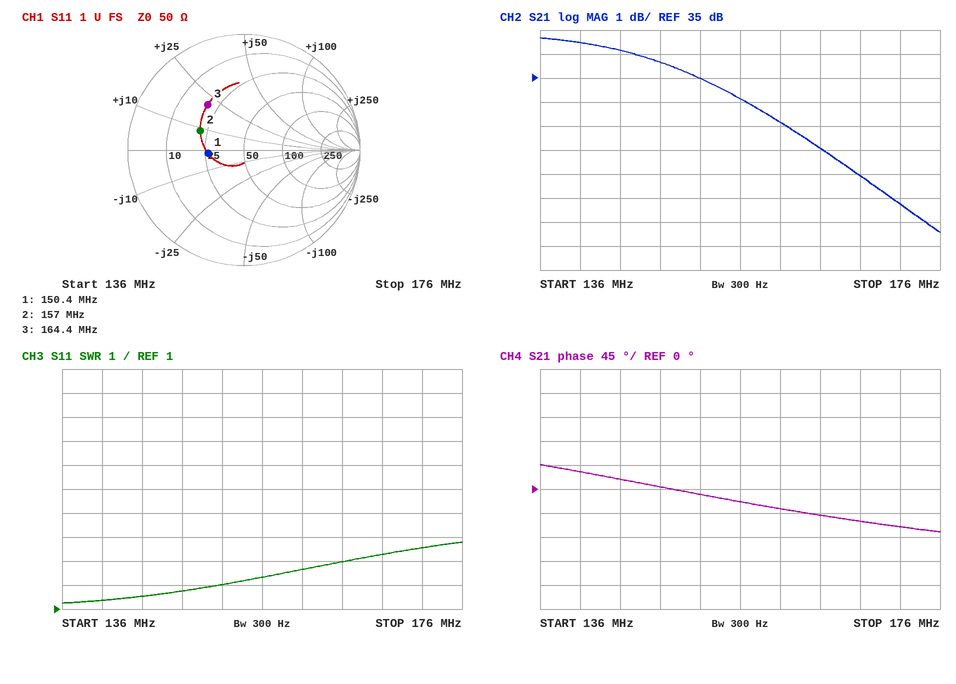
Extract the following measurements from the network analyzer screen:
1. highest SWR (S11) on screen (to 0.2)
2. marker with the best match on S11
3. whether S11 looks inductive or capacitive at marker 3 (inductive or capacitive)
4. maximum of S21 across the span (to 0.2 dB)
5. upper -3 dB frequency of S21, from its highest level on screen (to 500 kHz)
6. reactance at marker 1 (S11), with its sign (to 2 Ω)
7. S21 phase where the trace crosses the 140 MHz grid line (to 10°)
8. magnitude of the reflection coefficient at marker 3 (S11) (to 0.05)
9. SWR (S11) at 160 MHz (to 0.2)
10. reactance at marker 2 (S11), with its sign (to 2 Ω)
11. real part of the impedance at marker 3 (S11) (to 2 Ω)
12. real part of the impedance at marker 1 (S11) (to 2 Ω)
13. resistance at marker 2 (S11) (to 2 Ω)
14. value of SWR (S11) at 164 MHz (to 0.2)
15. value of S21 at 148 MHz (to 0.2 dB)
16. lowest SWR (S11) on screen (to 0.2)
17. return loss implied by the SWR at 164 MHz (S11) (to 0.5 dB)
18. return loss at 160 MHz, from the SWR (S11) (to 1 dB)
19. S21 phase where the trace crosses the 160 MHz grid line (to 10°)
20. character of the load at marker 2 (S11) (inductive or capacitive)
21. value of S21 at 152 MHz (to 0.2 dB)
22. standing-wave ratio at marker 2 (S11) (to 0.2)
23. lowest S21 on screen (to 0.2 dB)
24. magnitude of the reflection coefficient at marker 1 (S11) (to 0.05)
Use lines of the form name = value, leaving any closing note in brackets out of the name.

highest SWR (S11) on screen = 3.8
marker with the best match on S11 = marker 1
whether S11 looks inductive or capacitive at marker 3 = inductive
maximum of S21 across the span = 36.6 dB
upper -3 dB frequency of S21, from its highest level on screen = 158.0 MHz
reactance at marker 1 (S11), with its sign = -2 Ω
S21 phase where the trace crosses the 140 MHz grid line = 30°
magnitude of the reflection coefficient at marker 3 (S11) = 0.50
SWR (S11) at 160 MHz = 2.6
reactance at marker 2 (S11), with its sign = +8 Ω
real part of the impedance at marker 3 (S11) = 20 Ω
real part of the impedance at marker 1 (S11) = 26 Ω
resistance at marker 2 (S11) = 22 Ω
value of SWR (S11) at 164 MHz = 3.0
value of S21 at 148 MHz = 35.6 dB
lowest SWR (S11) on screen = 1.2
return loss implied by the SWR at 164 MHz (S11) = 6.0 dB
return loss at 160 MHz, from the SWR (S11) = 7 dB
S21 phase where the trace crosses the 160 MHz grid line = -40°
character of the load at marker 2 (S11) = inductive
value of S21 at 152 MHz = 35.0 dB
standing-wave ratio at marker 2 (S11) = 2.4
lowest S21 on screen = 28.6 dB
magnitude of the reflection coefficient at marker 1 (S11) = 0.30
